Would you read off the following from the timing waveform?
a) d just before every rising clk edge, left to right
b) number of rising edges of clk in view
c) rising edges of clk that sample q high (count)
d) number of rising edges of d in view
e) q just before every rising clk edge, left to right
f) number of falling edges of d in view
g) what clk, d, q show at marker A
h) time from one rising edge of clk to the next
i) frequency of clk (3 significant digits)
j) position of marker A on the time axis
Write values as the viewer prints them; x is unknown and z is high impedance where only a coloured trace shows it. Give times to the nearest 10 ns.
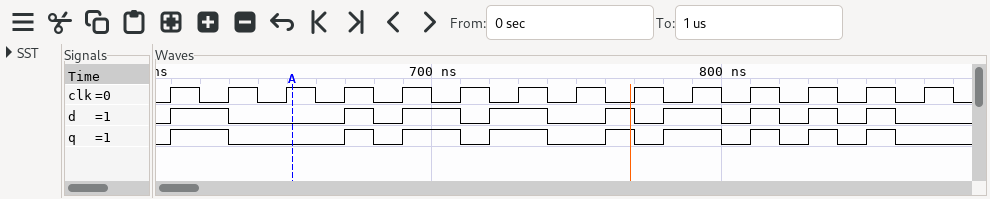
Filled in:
0 1 0 0 0 1 1 0 1 1 0 0 0 0
14
5
9
0 1 0 0 0 1 1 0 1 1 0 0 0 0
9
clk=1, d=0, q=0
20 ns
50.0 MHz
650 ns
